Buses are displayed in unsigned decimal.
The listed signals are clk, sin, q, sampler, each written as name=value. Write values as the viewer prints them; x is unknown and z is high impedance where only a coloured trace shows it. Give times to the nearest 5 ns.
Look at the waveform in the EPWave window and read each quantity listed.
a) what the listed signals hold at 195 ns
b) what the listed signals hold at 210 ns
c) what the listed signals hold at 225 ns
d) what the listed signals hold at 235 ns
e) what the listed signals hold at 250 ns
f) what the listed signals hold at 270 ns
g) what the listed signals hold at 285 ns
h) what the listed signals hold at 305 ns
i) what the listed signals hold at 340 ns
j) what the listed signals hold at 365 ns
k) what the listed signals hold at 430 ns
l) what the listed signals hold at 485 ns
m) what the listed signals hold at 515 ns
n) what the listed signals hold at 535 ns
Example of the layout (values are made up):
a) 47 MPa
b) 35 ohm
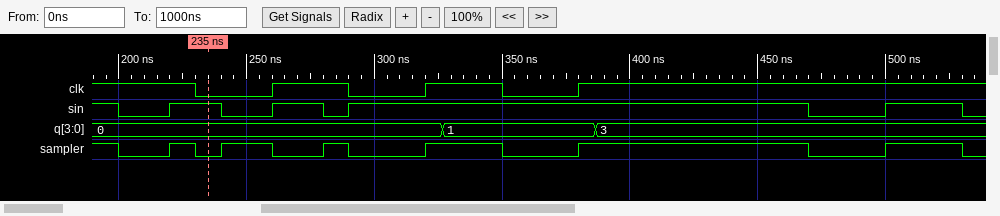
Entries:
a) clk=1, sin=1, q=0, sampler=1
b) clk=1, sin=0, q=0, sampler=0
c) clk=1, sin=1, q=0, sampler=1
d) clk=0, sin=1, q=0, sampler=0
e) clk=0, sin=0, q=0, sampler=1
f) clk=1, sin=1, q=0, sampler=0
g) clk=1, sin=0, q=0, sampler=1
h) clk=0, sin=1, q=0, sampler=0
i) clk=1, sin=1, q=1, sampler=1
j) clk=0, sin=1, q=1, sampler=0
k) clk=1, sin=1, q=3, sampler=1
l) clk=1, sin=0, q=3, sampler=0
m) clk=1, sin=1, q=3, sampler=1
n) clk=1, sin=0, q=3, sampler=0
